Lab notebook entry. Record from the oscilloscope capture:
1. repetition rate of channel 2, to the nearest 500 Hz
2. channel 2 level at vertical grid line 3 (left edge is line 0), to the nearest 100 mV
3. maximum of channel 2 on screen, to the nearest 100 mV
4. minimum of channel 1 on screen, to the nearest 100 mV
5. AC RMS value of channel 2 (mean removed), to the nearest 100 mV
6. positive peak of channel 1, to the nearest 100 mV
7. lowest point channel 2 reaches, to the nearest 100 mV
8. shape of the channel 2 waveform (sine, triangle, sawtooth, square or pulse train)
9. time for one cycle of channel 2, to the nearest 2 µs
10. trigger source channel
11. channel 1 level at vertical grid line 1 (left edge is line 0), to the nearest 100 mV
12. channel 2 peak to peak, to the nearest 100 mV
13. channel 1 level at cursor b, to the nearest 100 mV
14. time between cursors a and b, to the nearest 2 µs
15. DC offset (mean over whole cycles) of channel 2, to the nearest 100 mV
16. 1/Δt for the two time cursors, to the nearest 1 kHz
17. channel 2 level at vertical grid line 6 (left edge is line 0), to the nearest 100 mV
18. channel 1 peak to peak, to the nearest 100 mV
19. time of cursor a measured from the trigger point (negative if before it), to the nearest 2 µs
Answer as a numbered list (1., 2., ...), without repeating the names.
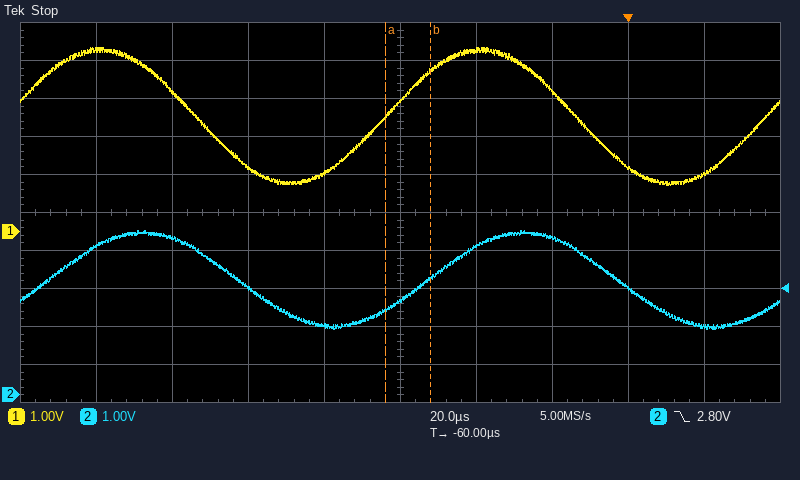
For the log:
1. 10.0 kHz
2. 2.8 V
3. 4.3 V
4. 1.2 V
5. 900 mV
6. 4.8 V
7. 1.7 V
8. sine
9. 100 µs
10. channel 2
11. 4.8 V
12. 2.6 V
13. 4.2 V
14. 12 µs
15. 3.0 V
16. 83 kHz
17. 3.9 V
18. 3.6 V
19. -64 µs
